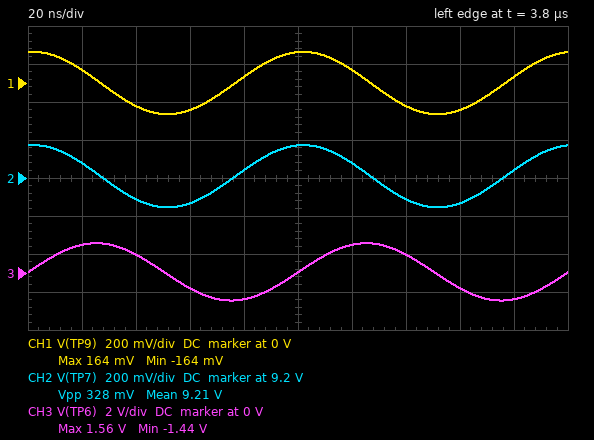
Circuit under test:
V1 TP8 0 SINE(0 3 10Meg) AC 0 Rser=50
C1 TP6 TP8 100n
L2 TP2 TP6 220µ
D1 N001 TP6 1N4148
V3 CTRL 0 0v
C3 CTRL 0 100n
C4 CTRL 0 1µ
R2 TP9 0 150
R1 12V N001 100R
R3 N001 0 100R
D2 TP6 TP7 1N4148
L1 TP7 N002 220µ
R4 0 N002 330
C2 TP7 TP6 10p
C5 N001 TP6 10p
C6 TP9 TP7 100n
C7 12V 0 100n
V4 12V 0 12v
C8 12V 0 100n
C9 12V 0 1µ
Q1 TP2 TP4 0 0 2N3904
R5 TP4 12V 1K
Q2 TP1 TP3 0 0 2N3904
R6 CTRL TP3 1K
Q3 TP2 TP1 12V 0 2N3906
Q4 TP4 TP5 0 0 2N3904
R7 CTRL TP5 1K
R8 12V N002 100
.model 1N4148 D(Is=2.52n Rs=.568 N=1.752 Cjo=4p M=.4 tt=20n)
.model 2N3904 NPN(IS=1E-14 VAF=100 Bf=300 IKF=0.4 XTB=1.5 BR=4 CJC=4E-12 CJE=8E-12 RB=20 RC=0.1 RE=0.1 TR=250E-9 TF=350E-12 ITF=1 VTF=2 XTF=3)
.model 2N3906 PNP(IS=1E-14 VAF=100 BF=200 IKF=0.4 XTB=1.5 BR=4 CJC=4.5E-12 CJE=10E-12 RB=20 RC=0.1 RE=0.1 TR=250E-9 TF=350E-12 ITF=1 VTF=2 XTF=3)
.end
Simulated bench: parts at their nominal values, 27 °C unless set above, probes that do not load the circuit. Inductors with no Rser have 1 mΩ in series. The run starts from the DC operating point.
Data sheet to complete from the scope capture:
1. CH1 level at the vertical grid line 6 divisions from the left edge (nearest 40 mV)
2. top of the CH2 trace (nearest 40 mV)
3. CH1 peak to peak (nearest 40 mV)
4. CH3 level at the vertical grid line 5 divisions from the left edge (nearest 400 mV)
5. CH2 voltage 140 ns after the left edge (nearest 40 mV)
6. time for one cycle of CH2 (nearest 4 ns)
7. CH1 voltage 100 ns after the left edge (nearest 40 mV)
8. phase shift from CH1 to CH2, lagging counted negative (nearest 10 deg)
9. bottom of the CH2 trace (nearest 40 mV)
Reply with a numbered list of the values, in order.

1. 80 mV
2. 9.36 V
3. 320 mV
4. 0 V
5. 9.08 V
6. 100 ns
7. 160 mV
8. 0 deg
9. 9.04 V
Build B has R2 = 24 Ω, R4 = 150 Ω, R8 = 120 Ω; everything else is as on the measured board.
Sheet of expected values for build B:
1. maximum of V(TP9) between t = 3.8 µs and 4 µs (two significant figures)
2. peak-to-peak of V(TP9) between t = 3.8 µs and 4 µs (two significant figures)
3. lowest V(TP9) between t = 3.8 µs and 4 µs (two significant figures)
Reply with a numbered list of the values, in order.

1. 27 mV
2. 54 mV
3. -27 mV
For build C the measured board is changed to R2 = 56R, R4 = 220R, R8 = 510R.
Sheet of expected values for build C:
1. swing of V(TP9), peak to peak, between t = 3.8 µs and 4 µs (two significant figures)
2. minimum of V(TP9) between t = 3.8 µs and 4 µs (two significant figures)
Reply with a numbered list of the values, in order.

1. 130 mV
2. -65 mV
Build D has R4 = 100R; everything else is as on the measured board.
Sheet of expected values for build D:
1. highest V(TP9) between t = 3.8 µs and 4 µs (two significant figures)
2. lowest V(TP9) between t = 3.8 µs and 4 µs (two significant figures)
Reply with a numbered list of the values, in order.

1. 170 mV
2. -170 mV
